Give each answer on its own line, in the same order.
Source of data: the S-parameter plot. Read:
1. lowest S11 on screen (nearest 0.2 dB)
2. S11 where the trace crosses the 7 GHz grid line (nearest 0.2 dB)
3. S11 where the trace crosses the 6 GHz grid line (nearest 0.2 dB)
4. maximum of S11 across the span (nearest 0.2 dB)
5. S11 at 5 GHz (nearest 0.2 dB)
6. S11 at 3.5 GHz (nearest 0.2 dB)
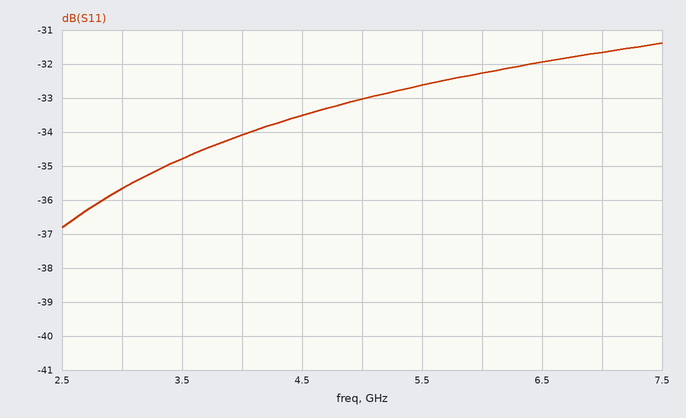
-36.8 dB
-31.6 dB
-32.2 dB
-31.4 dB
-33.0 dB
-34.8 dB
